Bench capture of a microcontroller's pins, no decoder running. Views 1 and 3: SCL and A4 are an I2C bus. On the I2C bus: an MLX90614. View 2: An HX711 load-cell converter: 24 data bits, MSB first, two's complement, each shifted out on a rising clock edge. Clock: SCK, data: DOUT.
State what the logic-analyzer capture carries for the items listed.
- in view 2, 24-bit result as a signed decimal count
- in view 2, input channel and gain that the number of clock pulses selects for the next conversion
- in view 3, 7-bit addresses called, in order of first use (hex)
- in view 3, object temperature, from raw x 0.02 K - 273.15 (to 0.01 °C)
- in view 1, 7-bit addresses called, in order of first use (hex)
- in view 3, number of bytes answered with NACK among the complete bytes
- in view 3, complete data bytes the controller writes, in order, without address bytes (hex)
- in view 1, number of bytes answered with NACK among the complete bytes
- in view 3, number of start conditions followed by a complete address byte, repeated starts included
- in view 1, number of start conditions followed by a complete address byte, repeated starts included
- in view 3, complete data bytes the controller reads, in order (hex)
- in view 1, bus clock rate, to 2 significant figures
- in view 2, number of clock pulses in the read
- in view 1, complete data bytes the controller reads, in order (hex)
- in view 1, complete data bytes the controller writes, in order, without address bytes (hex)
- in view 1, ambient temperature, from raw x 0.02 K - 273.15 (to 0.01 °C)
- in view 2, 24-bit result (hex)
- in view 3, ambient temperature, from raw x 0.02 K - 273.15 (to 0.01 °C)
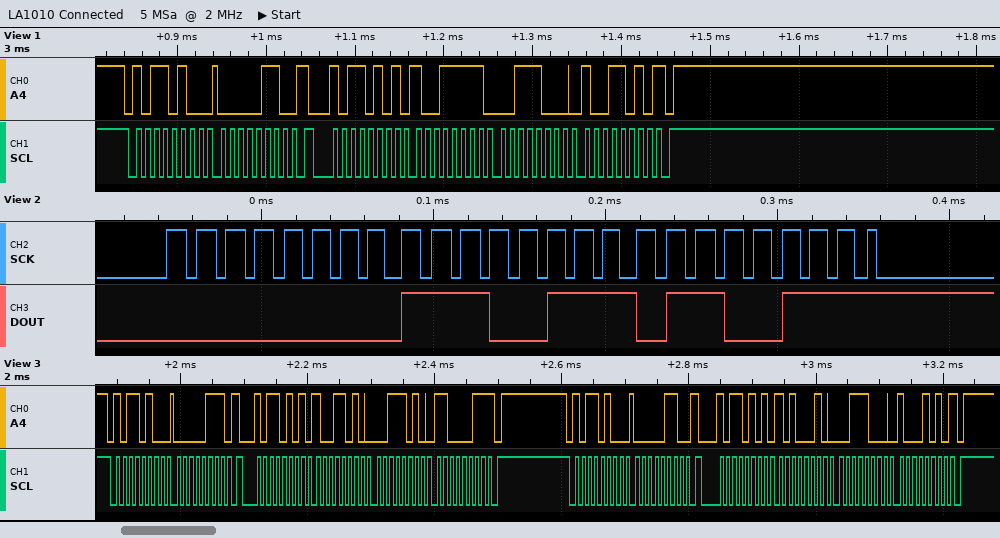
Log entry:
59239
channel A, gain 128
0x5A
26.89 °C
0x5A
2
07 06
1
4
2
9A 3A C3 A2 38 8A
100 kHz
25
9F 38 9A
06
16.75 °C
0x00E767
16.81 °C
